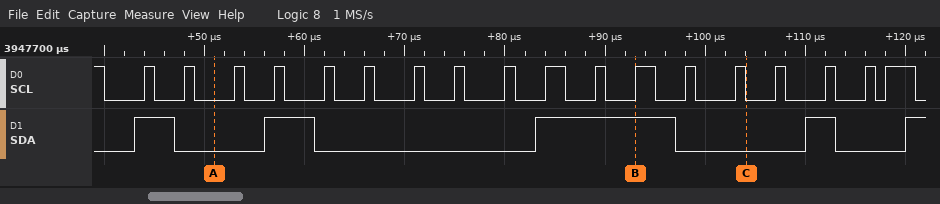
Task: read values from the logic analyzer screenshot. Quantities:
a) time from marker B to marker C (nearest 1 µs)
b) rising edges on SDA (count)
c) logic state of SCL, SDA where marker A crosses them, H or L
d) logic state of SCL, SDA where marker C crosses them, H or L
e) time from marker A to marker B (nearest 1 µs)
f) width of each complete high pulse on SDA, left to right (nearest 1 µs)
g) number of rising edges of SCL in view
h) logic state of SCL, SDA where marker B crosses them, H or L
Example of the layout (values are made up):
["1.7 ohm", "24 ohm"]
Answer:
["11 µs", "5", "SCL=L, SDA=L", "SCL=L, SDA=L", "42 µs", "4 µs, 5 µs, 14 µs, 3 µs", "18", "SCL=H, SDA=H"]
